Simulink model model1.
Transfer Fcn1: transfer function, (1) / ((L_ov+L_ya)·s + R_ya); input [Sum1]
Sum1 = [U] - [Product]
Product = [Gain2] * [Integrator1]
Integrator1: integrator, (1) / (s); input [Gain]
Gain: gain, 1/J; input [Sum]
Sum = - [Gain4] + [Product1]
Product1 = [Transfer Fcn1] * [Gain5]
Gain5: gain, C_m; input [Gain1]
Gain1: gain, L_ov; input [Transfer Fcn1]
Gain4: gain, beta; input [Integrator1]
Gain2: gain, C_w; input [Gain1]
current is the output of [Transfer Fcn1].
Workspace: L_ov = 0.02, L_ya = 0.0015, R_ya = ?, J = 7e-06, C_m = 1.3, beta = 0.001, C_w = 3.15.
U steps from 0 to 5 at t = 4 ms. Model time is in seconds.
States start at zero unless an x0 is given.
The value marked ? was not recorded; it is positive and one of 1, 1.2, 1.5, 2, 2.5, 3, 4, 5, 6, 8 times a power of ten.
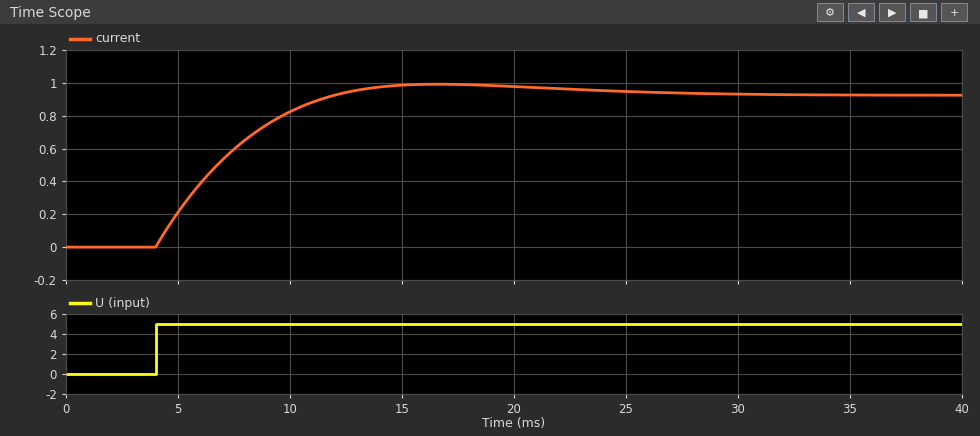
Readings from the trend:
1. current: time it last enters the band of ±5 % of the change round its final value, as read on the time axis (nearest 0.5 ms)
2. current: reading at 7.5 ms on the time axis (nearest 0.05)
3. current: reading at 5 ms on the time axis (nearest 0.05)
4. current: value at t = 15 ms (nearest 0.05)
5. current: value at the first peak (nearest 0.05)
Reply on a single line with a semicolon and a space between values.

21.0 ms; 0.60; 0.20; 1.00; 1.00
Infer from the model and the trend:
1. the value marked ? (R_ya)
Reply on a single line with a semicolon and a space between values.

4
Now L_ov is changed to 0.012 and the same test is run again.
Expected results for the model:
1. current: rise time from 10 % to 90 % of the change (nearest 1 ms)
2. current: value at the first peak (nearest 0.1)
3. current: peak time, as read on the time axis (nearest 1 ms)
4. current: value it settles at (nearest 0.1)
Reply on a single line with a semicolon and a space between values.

5 ms; 1.1; 15 ms; 1.1
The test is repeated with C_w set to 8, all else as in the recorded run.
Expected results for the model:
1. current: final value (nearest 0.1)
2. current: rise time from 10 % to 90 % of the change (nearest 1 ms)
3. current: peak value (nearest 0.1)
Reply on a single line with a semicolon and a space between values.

0.8; 4 ms; 0.9
